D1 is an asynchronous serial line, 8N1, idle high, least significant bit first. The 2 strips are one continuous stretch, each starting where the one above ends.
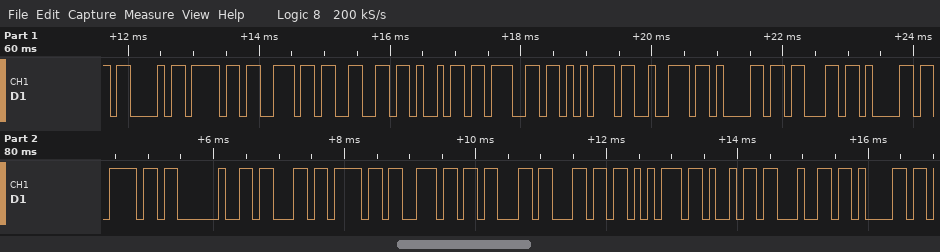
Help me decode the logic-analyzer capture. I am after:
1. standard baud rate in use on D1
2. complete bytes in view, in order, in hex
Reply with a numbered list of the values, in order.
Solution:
1. 9600 baud
2. 0x43 0x6F 0x6E 0x66 0x69 0x67 0x75 0x72 0x61 0x63 0x61 0x6F 0x20 0x63 0x6F 0x6E 0x63 0x6C 0x75 0x69 0x64 0x61
